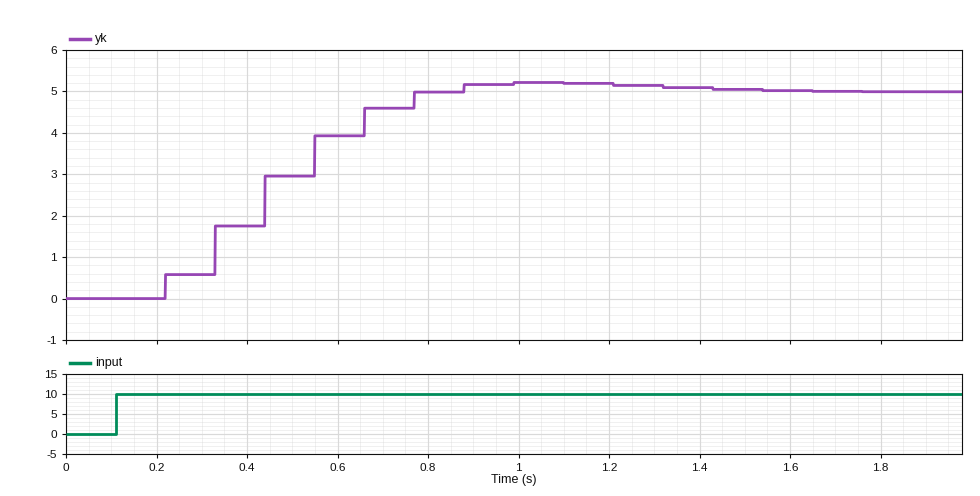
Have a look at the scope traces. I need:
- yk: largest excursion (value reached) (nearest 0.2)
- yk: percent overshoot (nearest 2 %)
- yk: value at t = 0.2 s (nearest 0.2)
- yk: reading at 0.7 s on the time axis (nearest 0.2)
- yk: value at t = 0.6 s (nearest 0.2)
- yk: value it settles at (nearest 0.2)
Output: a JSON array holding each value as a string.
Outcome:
["5.2", "4 %", "0.0", "4.6", "4.0", "5.0"]
